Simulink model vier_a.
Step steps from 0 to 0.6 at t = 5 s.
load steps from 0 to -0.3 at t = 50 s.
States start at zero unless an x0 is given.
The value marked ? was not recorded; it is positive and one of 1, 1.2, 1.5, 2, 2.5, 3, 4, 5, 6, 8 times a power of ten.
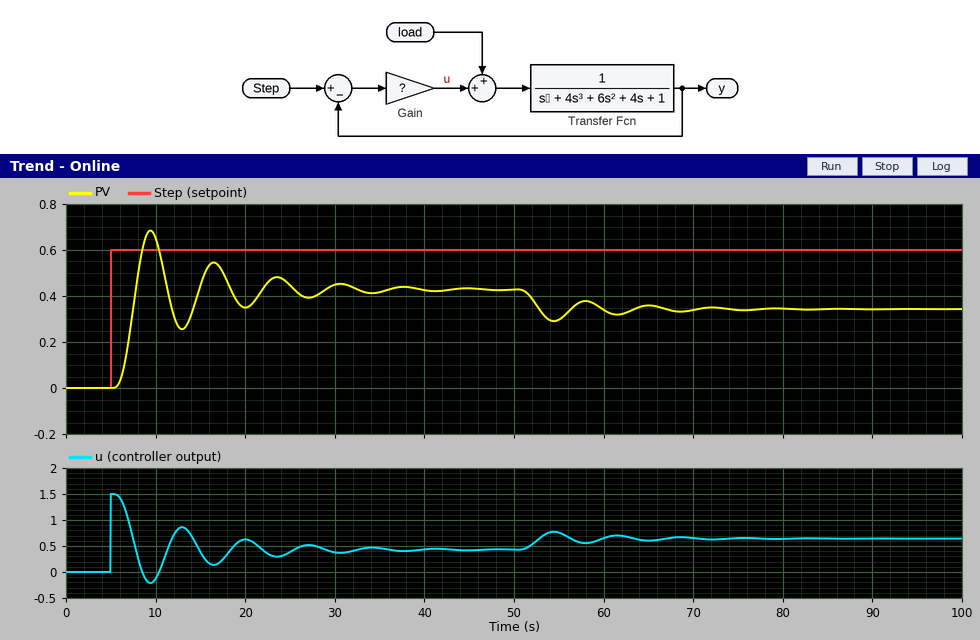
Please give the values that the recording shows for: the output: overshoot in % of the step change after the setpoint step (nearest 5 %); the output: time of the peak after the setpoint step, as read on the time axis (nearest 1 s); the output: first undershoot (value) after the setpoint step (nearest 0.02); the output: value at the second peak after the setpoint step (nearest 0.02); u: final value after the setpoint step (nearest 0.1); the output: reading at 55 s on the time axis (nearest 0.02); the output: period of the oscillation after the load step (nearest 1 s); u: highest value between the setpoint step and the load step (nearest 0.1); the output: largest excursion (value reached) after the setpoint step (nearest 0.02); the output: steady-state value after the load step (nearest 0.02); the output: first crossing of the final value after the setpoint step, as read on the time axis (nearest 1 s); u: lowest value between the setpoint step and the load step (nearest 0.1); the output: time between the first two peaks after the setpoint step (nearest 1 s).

60 %
9 s
0.26
0.54
0.4
0.30
7 s
1.5
0.68
0.34
8 s
-0.2
7 s
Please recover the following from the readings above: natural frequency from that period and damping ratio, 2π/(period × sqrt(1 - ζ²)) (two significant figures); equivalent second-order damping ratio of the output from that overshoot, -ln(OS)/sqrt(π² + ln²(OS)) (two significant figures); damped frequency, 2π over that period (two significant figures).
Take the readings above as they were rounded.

0.91 rad/s
0.16
0.90 rad/s
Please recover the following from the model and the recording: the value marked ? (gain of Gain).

2.5
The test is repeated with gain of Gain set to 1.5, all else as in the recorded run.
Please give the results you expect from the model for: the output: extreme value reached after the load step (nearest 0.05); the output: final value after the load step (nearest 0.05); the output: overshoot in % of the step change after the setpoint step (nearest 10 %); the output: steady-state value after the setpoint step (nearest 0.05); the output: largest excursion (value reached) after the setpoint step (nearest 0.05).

0.20
0.25
40 %
0.35
0.50
